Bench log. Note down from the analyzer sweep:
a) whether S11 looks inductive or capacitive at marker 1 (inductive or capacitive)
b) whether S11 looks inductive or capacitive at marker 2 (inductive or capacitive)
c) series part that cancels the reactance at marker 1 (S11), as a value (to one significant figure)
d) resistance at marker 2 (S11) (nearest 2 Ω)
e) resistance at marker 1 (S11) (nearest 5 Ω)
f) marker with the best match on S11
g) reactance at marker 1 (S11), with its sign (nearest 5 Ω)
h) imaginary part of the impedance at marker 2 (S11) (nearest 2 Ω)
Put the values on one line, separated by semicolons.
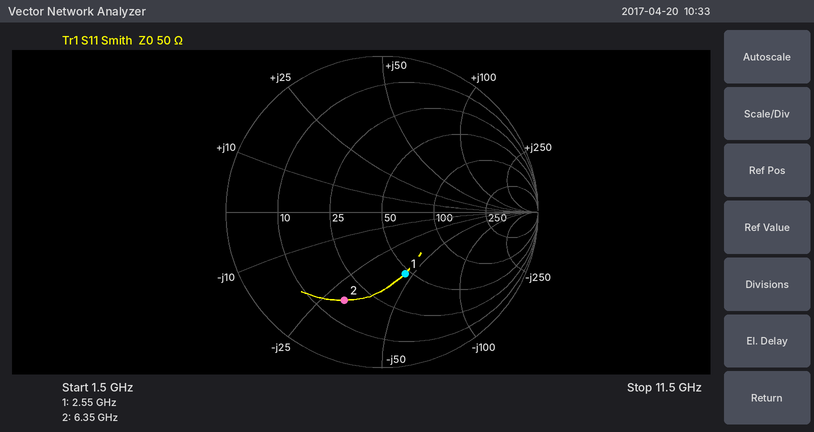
capacitive; capacitive; 3 nH; 16 Ω; 45 Ω; marker 1; -45 Ω; -30 Ω
